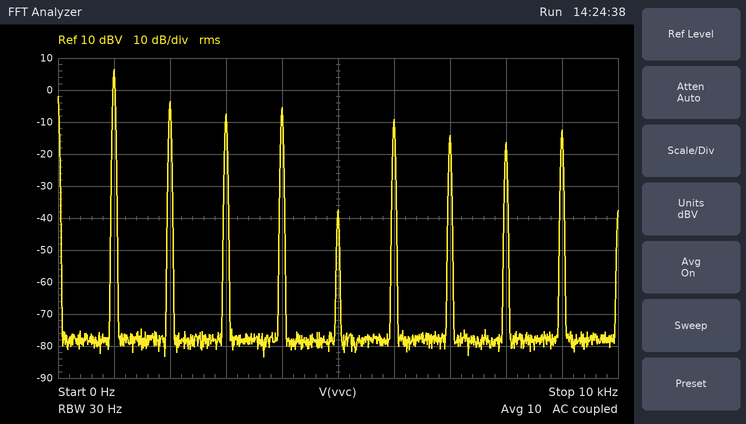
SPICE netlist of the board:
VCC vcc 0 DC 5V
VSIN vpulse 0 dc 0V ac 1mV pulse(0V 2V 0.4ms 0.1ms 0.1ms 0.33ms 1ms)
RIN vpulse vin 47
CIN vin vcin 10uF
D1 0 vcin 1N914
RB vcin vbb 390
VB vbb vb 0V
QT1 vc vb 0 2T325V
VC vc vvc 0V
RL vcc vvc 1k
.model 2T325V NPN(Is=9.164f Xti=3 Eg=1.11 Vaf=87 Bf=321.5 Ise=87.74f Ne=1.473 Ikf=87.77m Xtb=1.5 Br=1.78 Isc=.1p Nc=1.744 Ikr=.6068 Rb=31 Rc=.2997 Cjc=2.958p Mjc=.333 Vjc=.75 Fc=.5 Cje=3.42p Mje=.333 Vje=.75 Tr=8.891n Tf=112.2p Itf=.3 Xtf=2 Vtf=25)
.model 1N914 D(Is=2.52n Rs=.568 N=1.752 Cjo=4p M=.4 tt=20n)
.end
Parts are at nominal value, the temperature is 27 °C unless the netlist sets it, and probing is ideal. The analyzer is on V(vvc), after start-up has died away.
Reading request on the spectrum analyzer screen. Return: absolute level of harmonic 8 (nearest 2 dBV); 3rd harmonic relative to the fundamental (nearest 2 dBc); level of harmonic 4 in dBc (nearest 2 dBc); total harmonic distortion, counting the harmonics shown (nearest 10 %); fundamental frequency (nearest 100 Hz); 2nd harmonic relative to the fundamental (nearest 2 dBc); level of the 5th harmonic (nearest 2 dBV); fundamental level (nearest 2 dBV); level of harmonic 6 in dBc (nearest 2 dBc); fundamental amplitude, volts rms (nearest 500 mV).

-16 dBV
-14 dBc
-12 dBc
50 %
1.0 kHz
-10 dBc
-38 dBV
6 dBV
-16 dBc
2.0 V
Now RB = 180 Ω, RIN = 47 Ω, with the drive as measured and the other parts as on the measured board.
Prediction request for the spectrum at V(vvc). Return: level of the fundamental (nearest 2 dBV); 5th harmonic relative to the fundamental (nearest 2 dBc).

6 dBV
-32 dBc
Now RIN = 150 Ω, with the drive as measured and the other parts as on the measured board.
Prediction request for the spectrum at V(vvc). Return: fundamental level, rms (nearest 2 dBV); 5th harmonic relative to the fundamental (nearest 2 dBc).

6 dBV
-32 dBc
